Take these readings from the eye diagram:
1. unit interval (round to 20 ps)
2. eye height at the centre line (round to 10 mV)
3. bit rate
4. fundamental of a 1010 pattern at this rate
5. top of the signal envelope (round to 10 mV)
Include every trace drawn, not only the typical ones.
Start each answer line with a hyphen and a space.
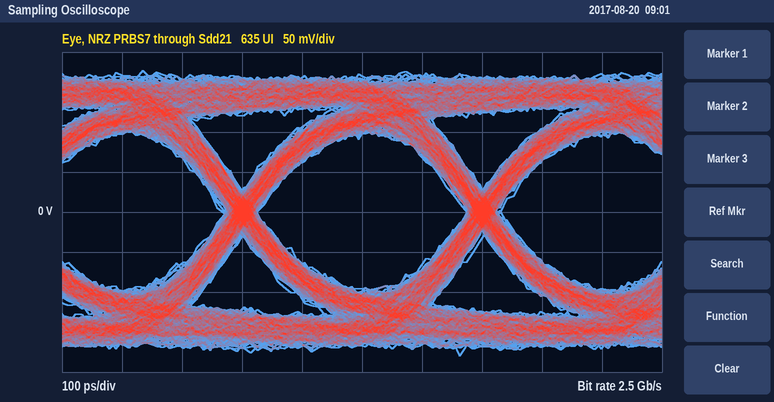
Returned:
- 400 ps
- 190 mV
- 2.5 Gb/s
- 1.25 GHz
- 180 mV
